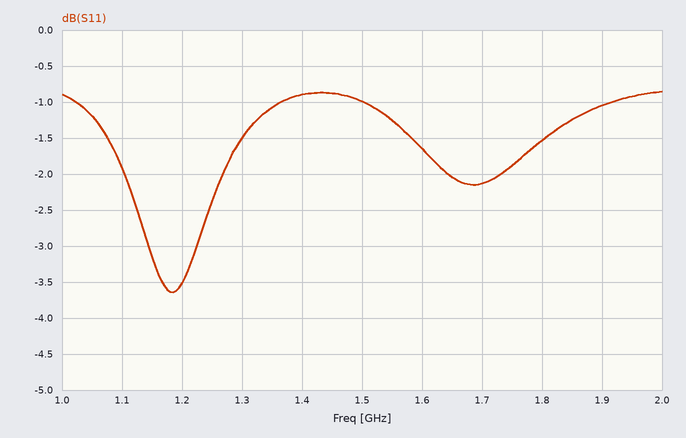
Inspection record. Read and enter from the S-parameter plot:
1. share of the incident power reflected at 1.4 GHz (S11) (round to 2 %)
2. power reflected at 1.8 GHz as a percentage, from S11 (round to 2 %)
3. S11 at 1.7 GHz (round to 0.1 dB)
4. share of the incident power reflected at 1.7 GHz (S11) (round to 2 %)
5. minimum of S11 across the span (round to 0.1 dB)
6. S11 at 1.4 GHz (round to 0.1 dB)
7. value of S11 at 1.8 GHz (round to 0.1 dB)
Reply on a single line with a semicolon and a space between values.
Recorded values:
82 %; 70 %; -2.1 dB; 62 %; -3.6 dB; -0.9 dB; -1.5 dB
